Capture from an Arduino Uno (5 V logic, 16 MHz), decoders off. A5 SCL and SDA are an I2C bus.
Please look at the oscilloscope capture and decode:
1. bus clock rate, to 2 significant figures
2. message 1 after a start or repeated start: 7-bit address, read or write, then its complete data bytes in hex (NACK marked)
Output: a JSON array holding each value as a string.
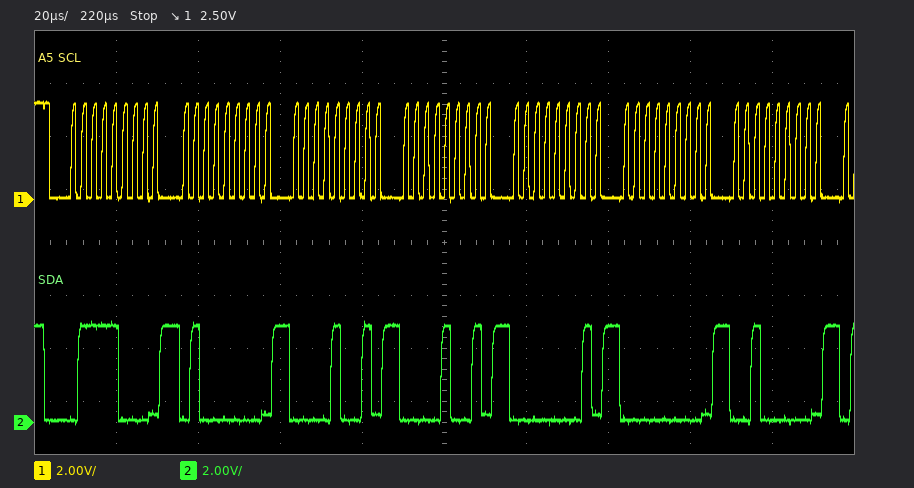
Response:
["400 kHz", "0x3C write: 40 09 09 01 00 20"]
